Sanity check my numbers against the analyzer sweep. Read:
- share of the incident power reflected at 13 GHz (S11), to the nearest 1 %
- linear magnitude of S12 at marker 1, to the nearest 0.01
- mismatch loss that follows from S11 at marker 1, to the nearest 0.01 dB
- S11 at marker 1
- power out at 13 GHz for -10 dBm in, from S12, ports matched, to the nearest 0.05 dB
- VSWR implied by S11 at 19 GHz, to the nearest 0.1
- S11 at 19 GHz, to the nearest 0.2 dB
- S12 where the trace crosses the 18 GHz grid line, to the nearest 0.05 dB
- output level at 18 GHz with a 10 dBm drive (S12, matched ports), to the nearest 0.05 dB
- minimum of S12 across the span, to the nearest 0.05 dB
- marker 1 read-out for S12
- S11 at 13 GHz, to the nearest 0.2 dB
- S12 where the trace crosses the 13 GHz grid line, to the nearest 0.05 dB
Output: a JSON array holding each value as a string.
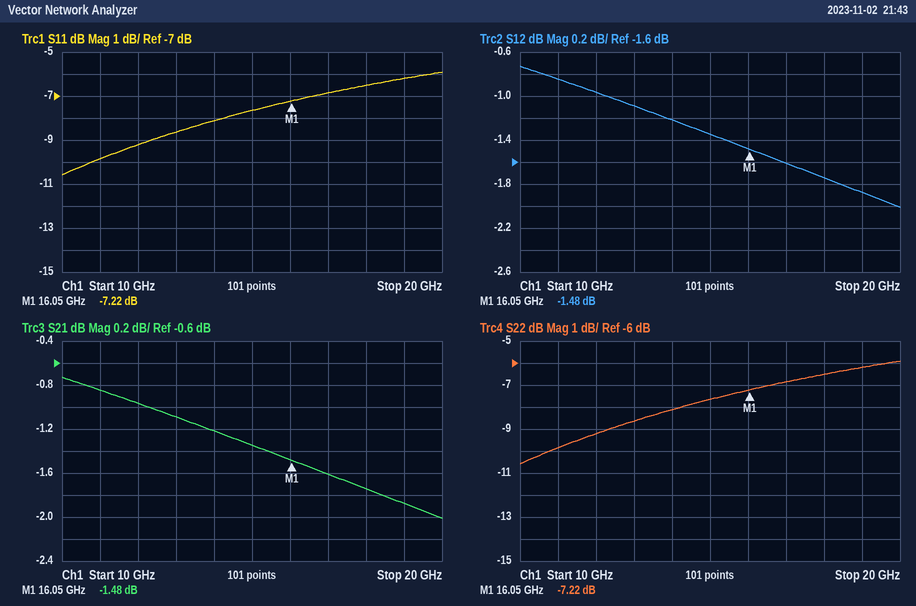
["14 %", "0.84", "0.91 dB", "-7.22 dB", "-11.10 dBm", "2.9", "-6.2 dB", "-1.75 dB", "8.25 dBm", "-2.00 dB", "-1.48 dB", "-8.6 dB", "-1.10 dB"]
